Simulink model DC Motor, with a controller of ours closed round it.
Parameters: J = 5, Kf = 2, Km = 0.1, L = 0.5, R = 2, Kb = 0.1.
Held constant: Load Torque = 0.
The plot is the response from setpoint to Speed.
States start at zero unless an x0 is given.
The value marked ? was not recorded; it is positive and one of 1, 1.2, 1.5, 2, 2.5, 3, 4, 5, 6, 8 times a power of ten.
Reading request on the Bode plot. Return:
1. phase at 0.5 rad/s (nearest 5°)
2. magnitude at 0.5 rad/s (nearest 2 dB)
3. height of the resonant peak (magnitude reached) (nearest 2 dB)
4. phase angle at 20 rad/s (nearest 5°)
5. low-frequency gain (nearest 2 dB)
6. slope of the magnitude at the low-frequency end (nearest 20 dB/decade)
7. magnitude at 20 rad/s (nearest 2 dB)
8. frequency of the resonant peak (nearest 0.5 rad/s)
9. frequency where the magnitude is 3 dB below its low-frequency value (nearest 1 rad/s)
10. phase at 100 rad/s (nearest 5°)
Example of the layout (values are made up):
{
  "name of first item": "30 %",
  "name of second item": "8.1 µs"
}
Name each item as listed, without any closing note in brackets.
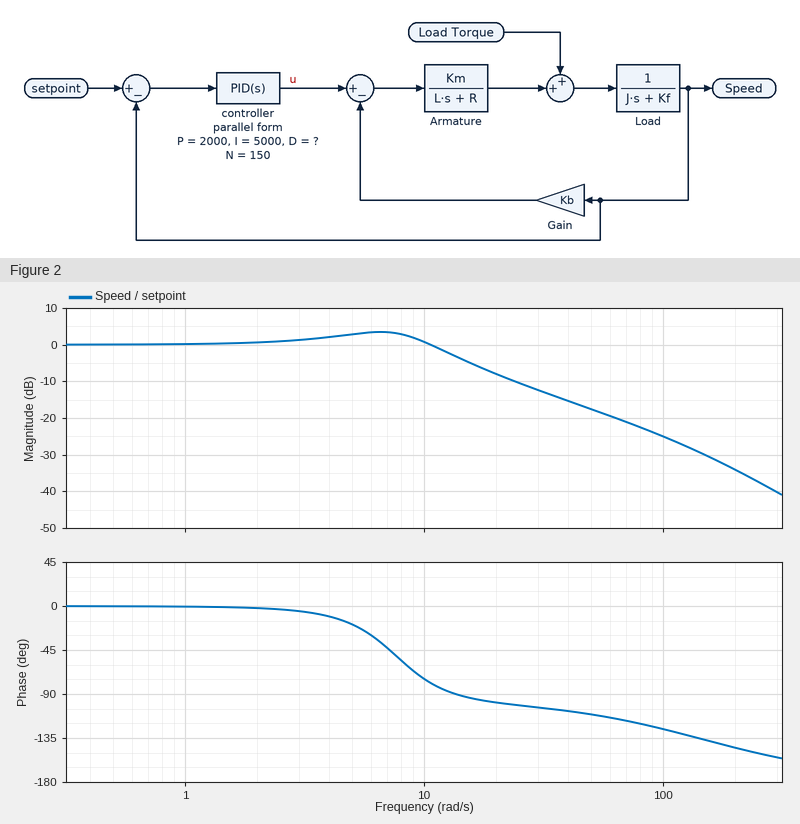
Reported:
{
  "phase at 0.5 rad/s": "0°",
  "magnitude at 0.5 rad/s": "0 dB",
  "height of the resonant peak (magnitude reached)": "4 dB",
  "phase angle at 20 rad/s": "-100°",
  "low-frequency gain": "0 dB",
  "slope of the magnitude at the low-frequency end": "0 dB/decade",
  "magnitude at 20 rad/s": "-8 dB",
  "frequency of the resonant peak": "6.5 rad/s",
  "frequency where the magnitude is 3 dB below its low-frequency value": "13 rad/s",
  "phase at 100 rad/s": "-125°"
}
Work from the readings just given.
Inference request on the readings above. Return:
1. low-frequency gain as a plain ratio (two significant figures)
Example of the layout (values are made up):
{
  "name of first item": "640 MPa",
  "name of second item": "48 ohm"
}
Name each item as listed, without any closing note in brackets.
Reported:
{
  "low-frequency gain as a plain ratio": "1.0"
}
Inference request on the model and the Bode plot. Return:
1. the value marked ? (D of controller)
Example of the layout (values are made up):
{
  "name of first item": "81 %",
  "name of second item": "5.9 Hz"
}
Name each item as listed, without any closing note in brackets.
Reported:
{
  "the value marked ?": "150"
}
